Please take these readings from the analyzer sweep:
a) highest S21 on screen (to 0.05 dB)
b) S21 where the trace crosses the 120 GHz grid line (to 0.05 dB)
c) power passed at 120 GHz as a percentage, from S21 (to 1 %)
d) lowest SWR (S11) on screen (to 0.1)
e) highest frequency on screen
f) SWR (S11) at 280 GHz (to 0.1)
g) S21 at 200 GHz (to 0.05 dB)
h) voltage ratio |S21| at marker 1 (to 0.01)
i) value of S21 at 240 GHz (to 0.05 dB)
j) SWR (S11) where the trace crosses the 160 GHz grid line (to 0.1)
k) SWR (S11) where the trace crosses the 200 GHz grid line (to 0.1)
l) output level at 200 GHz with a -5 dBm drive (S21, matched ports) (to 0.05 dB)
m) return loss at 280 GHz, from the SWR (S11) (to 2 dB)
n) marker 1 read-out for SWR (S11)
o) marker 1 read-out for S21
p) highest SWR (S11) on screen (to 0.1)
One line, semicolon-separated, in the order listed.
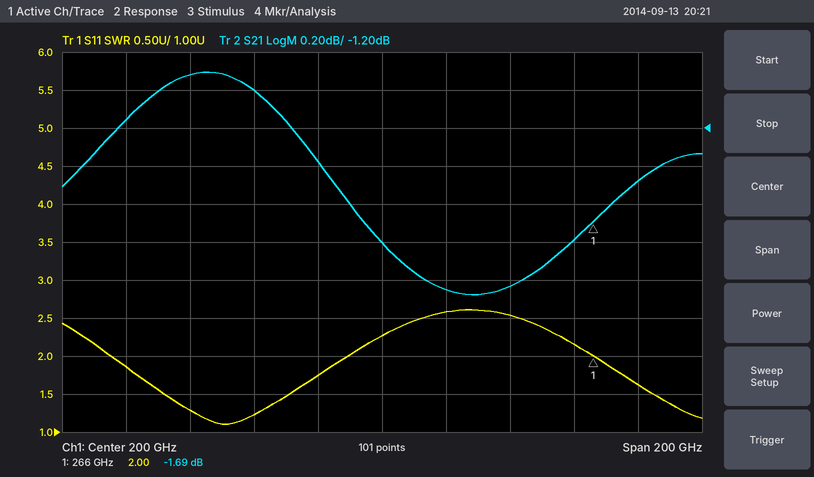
-0.90 dB; -1.15 dB; 77 %; 1.1; 300 GHz; 1.6; -1.80 dB; 0.82; -2.05 dB; 1.2; 2.3; -6.80 dBm; 12 dB; 2.00; -1.69 dB; 2.6
